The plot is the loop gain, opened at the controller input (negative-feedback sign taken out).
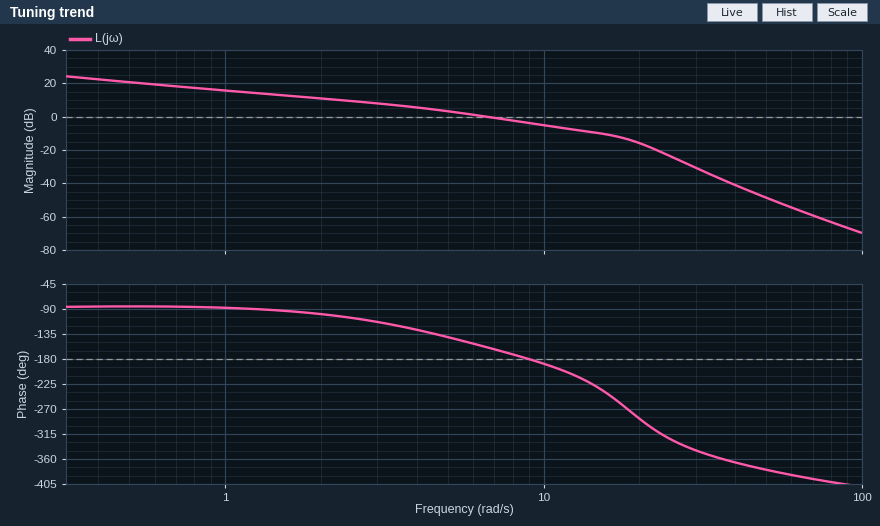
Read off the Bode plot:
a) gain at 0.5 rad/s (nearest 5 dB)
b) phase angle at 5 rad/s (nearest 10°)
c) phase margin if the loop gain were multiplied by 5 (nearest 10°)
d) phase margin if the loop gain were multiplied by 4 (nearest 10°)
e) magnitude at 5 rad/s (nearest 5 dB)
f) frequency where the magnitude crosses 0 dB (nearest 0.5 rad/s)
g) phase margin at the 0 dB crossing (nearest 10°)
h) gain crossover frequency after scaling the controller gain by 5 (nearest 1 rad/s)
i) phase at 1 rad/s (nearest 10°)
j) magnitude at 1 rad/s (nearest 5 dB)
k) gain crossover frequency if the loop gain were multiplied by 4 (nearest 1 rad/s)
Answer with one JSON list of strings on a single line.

["20 dB", "-140°", "-90°", "-80°", "5 dB", "6.5 rad/s", "20°", "19 rad/s", "-90°", "15 dB", "17 rad/s"]
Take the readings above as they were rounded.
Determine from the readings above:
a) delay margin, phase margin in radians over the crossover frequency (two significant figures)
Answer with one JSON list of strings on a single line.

["0.054 s"]
